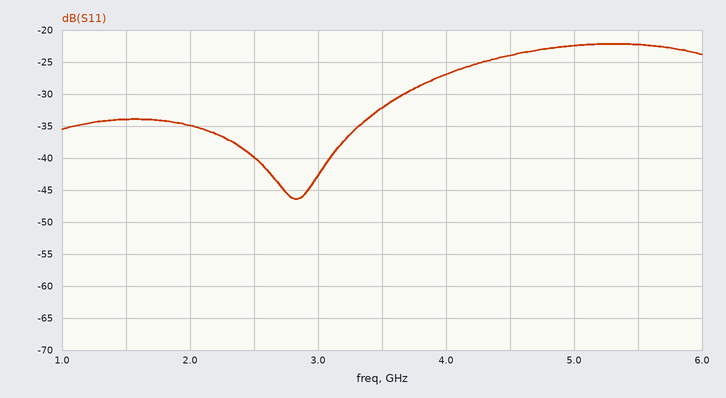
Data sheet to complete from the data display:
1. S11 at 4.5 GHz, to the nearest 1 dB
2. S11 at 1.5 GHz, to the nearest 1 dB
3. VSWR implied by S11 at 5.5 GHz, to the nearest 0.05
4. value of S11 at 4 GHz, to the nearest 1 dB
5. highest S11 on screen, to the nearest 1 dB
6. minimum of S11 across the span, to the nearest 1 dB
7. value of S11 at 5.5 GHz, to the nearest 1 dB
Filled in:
-24 dB
-34 dB
1.15
-27 dB
-22 dB
-46 dB
-22 dB
